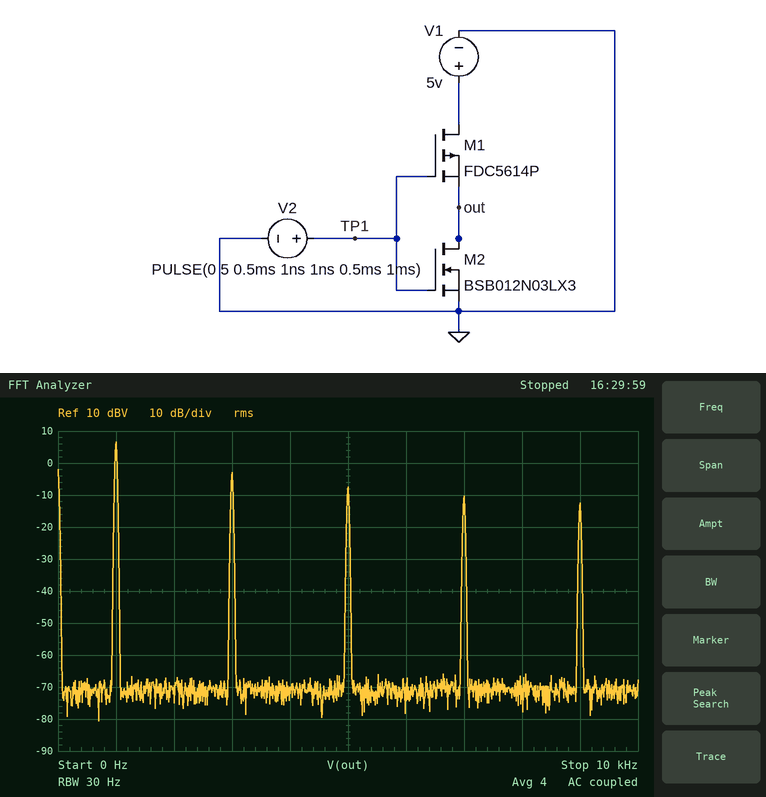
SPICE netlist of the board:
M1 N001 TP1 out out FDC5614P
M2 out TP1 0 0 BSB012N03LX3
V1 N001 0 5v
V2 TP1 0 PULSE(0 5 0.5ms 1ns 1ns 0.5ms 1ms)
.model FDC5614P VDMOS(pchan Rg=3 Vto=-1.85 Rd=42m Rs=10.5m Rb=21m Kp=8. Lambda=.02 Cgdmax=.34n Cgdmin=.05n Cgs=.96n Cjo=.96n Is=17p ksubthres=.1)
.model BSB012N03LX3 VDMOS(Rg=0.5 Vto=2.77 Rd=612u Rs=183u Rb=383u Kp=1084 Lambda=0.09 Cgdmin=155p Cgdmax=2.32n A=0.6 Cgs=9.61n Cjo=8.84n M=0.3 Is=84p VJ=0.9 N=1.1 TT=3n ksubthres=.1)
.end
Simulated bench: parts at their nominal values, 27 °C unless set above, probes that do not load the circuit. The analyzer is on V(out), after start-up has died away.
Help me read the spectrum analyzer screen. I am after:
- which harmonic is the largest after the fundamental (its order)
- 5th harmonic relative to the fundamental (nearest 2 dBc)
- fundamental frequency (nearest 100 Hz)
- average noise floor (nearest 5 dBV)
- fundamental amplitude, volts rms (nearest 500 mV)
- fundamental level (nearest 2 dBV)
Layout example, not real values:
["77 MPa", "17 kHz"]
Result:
["3", "-14 dBc", "1.0 kHz", "-70 dBV", "2.0 V", "6 dBV"]
